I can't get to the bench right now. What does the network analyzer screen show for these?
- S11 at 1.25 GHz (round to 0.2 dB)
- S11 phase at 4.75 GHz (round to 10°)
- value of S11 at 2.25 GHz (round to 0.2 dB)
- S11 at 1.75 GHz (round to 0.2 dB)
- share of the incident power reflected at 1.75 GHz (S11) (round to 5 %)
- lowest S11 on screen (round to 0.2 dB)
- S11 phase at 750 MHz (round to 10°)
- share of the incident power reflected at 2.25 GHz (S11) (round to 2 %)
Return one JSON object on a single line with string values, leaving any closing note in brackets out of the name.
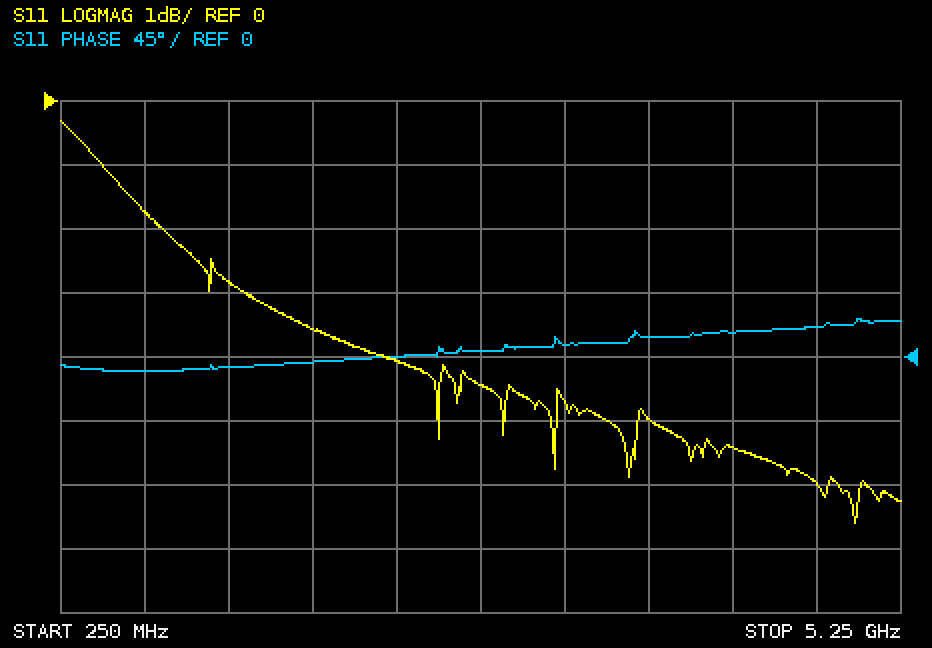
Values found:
{"S11 at 1.25 GHz": "-2.8 dB", "S11 phase at 4.75 GHz": "20°", "value of S11 at 2.25 GHz": "-4.0 dB", "S11 at 1.75 GHz": "-3.6 dB", "share of the incident power reflected at 1.75 GHz (S11)": "45 %", "lowest S11 on screen": "-6.6 dB", "S11 phase at 750 MHz": "-10°", "share of the incident power reflected at 2.25 GHz (S11)": "40 %"}
